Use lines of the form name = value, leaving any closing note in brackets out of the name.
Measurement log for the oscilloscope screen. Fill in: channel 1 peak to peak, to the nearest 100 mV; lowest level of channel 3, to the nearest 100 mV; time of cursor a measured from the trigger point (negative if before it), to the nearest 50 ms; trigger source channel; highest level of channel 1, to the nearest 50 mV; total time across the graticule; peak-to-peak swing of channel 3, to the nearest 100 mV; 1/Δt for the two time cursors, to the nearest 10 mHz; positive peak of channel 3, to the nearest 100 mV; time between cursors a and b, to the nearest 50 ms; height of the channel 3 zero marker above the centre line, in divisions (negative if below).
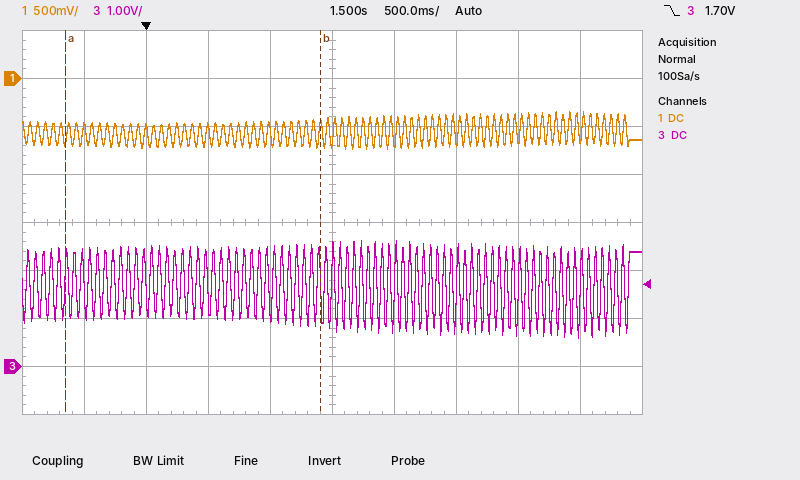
channel 1 peak to peak, to the nearest 100 mV = 400 mV
lowest level of channel 3, to the nearest 100 mV = 600 mV
time of cursor a measured from the trigger point (negative if before it), to the nearest 50 ms = -650 ms
trigger source channel = channel 3
highest level of channel 1, to the nearest 50 mV = -350 mV
total time across the graticule = 5 s
peak-to-peak swing of channel 3, to the nearest 100 mV = 2.0 V
1/Δt for the two time cursors, to the nearest 10 mHz = 490 mHz
positive peak of channel 3, to the nearest 100 mV = 2.6 V
time between cursors a and b, to the nearest 50 ms = 2.05 s
height of the channel 3 zero marker above the centre line, in divisions = -3.0 div
